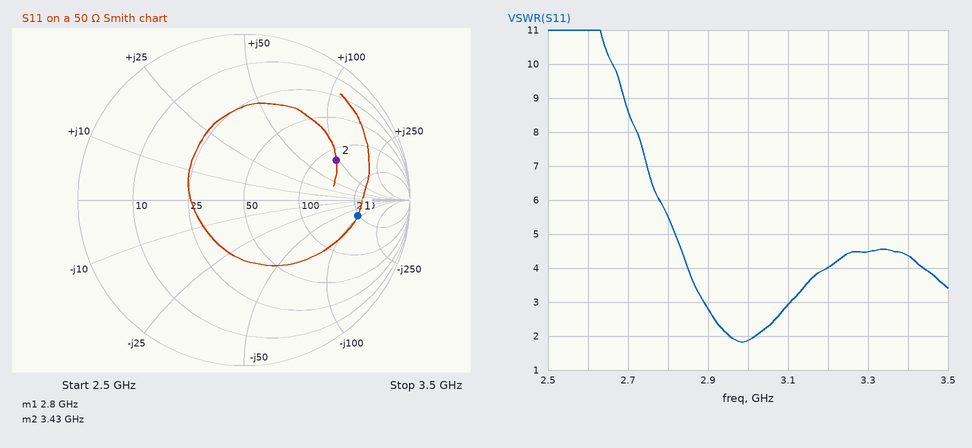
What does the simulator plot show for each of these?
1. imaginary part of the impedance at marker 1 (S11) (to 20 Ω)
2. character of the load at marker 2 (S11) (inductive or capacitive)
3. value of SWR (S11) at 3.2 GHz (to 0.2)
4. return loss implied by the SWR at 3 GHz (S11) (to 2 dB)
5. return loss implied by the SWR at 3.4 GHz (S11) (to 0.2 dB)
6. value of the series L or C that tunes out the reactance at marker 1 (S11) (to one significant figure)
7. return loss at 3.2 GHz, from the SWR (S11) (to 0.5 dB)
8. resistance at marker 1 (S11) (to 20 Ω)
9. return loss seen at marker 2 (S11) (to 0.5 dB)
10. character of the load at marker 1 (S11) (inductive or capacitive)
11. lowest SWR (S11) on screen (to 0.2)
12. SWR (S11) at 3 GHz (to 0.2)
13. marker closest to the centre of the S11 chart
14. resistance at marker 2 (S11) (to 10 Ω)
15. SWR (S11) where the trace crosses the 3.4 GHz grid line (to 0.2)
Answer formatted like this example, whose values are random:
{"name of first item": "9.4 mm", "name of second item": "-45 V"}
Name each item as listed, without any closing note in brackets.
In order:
{"imaginary part of the impedance at marker 1 (S11)": "-80 Ω", "character of the load at marker 2 (S11)": "inductive", "value of SWR (S11) at 3.2 GHz": "4.0", "return loss implied by the SWR at 3 GHz (S11)": "10 dB", "return loss implied by the SWR at 3.4 GHz (S11)": "4.0 dB", "value of the series L or C that tunes out the reactance at marker 1 (S11)": "5 nH", "return loss at 3.2 GHz, from the SWR (S11)": "4.5 dB", "resistance at marker 1 (S11)": "240 Ω", "return loss seen at marker 2 (S11)": "4.5 dB", "character of the load at marker 1 (S11)": "capacitive", "lowest SWR (S11) on screen": "1.8", "SWR (S11) at 3 GHz": "1.8", "marker closest to the centre of the S11 chart": "marker 2", "resistance at marker 2 (S11)": "120 Ω", "SWR (S11) where the trace crosses the 3.4 GHz grid line": "4.4"}
